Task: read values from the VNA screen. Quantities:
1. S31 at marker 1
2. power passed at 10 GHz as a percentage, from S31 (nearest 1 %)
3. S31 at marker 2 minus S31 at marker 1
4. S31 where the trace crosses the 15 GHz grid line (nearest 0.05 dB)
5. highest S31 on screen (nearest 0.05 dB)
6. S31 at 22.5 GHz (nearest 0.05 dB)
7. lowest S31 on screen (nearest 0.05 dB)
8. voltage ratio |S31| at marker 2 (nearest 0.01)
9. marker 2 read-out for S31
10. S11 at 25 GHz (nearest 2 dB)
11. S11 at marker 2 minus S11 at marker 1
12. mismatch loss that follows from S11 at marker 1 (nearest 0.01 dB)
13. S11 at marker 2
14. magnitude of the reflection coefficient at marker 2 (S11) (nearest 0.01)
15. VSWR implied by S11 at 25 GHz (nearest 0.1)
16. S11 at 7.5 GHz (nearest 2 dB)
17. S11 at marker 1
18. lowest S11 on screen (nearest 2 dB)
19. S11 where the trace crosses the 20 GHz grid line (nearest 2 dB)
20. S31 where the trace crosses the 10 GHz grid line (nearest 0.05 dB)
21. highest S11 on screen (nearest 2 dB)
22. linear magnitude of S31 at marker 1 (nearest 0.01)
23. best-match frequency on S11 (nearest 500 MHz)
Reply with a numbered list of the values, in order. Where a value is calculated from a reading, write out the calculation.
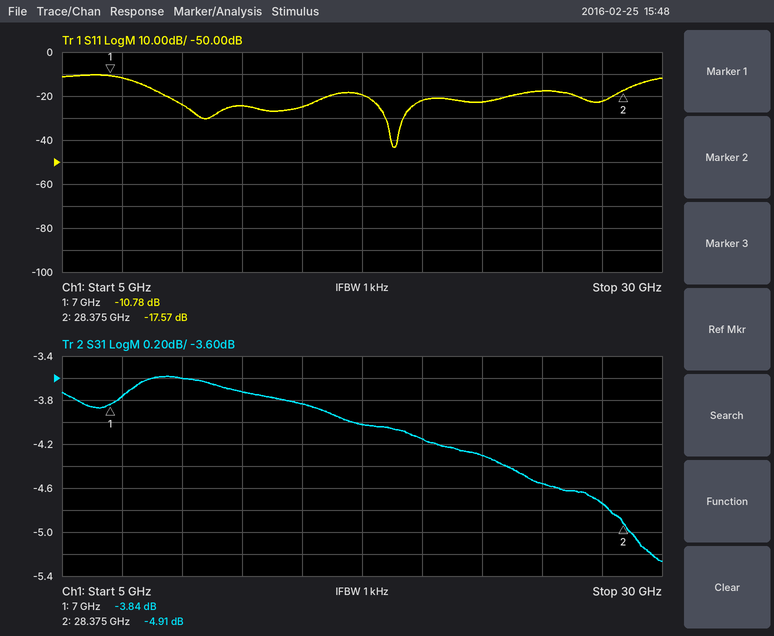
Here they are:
1. -3.84 dB
2. 10^(-3.6/10) ≈ 44 %
3. -4.91 − (-3.84) = -1.07 dB
4. -3.85 dB
5. -3.60 dB
6. -4.30 dB
7. -5.25 dB
8. 10^(-4.91/20) ≈ 0.57
9. -4.91 dB
10. -18 dB
11. -17.57 − (-10.78) = -6.79 dB
12. −10 log10(1 − 10^(-10.78/10)) ≈ 0.38 dB
13. -17.57 dB
14. 10^(-17.57/20) ≈ 0.13
15. |Γ| = 10^(-18/20) = 0.1259; VSWR = (1 + 0.1259)/(1 − 0.1259) ≈ 1.3
16. -12 dB
17. -10.78 dB
18. -44 dB
19. -22 dB
20. -3.60 dB
21. -10 dB
22. 10^(-3.84/20) ≈ 0.64
23. 19.0 GHz
